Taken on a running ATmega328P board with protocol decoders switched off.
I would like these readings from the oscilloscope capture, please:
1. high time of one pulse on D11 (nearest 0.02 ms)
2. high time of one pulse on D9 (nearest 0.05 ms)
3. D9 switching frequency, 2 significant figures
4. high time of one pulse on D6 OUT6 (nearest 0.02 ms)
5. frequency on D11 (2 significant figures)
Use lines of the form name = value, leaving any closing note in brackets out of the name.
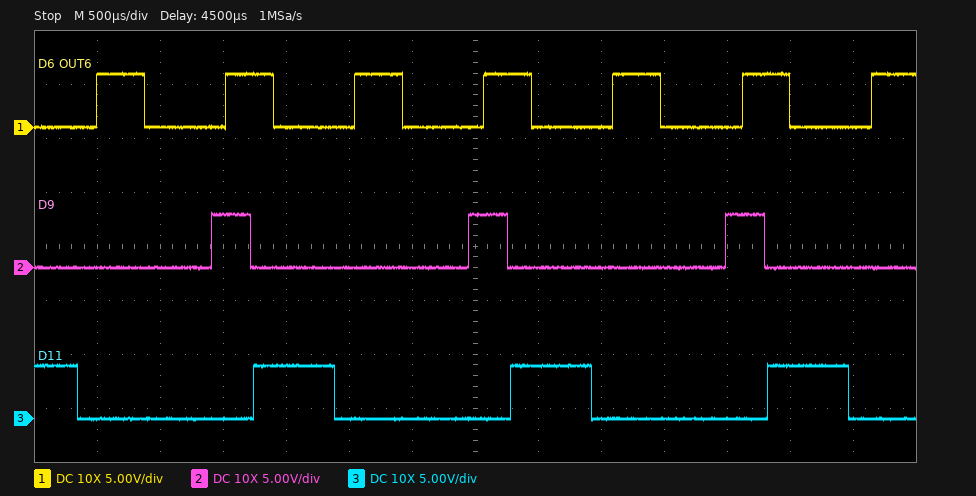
high time of one pulse on D11 = 0.64 ms
high time of one pulse on D9 = 0.30 ms
D9 switching frequency, 2 significant figures = 490 Hz
high time of one pulse on D6 OUT6 = 0.38 ms
frequency on D11 = 490 Hz
